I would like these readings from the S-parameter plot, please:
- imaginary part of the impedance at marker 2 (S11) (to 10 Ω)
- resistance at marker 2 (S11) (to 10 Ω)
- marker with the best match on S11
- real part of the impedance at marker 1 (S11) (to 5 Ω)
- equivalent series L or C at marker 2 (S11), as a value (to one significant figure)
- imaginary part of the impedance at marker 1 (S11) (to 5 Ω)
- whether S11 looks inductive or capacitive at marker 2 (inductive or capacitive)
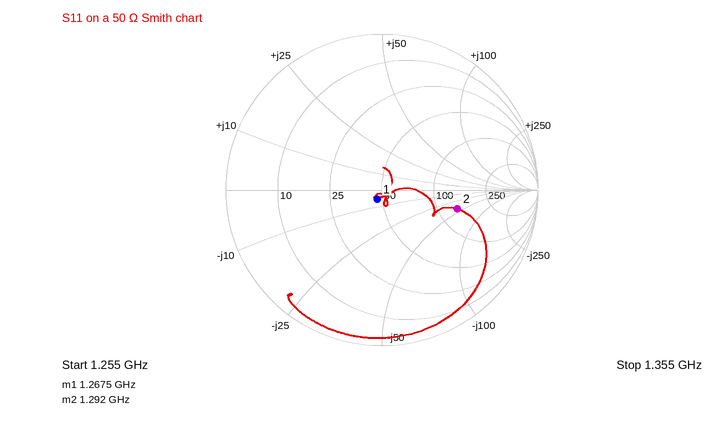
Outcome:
-40 Ω
130 Ω
marker 1
45 Ω
3 pF
-5 Ω
capacitive
